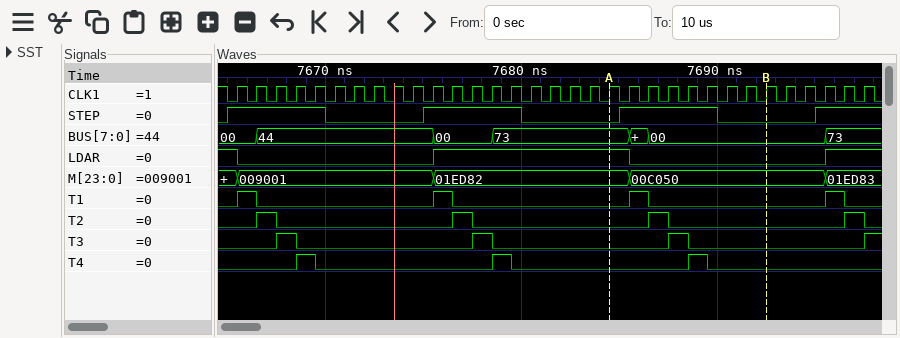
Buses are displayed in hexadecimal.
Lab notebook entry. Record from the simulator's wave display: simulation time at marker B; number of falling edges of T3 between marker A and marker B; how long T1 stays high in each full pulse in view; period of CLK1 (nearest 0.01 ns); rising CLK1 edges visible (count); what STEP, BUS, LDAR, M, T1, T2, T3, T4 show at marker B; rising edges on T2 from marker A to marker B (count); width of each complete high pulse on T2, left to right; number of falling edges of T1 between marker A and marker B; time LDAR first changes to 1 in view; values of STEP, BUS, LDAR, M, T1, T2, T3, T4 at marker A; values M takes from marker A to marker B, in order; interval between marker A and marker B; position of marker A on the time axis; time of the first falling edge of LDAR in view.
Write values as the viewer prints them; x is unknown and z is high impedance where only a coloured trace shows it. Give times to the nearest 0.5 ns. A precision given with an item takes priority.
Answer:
7692.5 ns
1
1 ns, 1 ns, 1 ns, 1 ns
1 ns
33
STEP=0, BUS=00, LDAR=0, M=00C050, T1=0, T2=0, T3=0, T4=0
1
1 ns, 1 ns, 1 ns, 1 ns
1
7675.5 ns
STEP=0, BUS=73, LDAR=1, M=01ED82, T1=0, T2=0, T3=0, T4=0
01ED82, 00C050
8 ns
7684.5 ns
7665.5 ns
